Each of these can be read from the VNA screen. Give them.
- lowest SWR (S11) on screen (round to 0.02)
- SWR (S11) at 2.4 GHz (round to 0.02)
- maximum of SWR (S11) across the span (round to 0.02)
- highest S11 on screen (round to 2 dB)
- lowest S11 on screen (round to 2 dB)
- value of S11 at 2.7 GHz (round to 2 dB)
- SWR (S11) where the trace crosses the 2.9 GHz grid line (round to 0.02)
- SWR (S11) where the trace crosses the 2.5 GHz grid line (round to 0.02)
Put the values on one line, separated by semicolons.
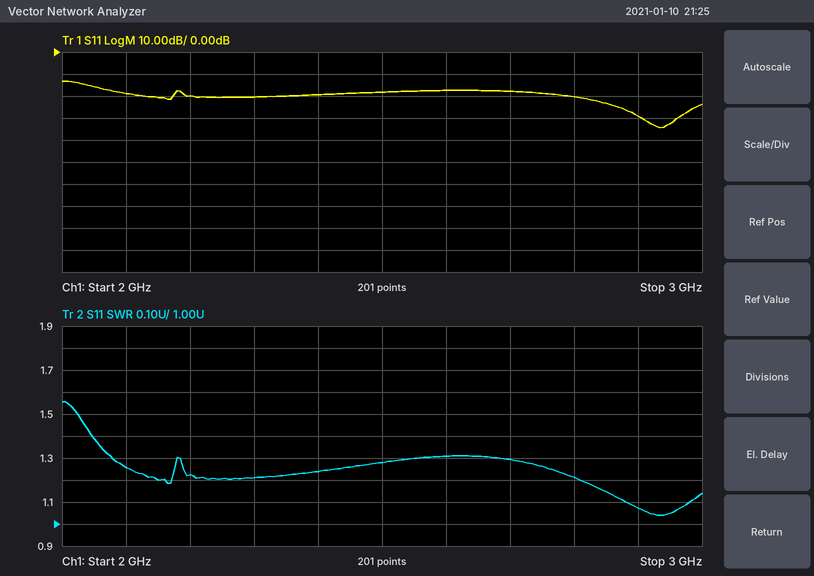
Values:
1.04; 1.24; 1.56; -14 dB; -34 dB; -18 dB; 1.08; 1.28
